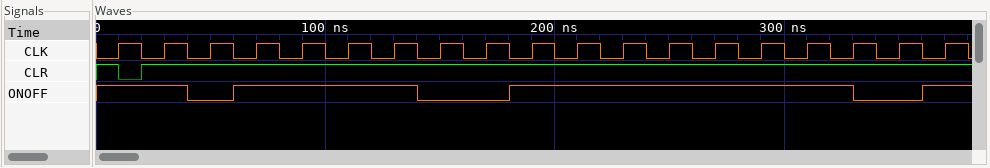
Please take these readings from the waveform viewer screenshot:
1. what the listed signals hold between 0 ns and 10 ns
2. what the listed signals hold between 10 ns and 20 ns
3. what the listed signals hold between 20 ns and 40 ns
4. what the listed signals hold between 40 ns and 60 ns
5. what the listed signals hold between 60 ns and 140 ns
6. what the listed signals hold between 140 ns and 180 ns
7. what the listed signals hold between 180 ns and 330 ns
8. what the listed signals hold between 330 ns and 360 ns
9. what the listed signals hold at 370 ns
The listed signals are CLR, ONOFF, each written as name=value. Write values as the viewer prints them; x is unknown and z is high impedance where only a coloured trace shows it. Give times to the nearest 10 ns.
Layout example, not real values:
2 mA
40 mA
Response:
CLR=1, ONOFF=1
CLR=0, ONOFF=1
CLR=1, ONOFF=1
CLR=1, ONOFF=0
CLR=1, ONOFF=1
CLR=1, ONOFF=0
CLR=1, ONOFF=1
CLR=1, ONOFF=0
CLR=1, ONOFF=1
